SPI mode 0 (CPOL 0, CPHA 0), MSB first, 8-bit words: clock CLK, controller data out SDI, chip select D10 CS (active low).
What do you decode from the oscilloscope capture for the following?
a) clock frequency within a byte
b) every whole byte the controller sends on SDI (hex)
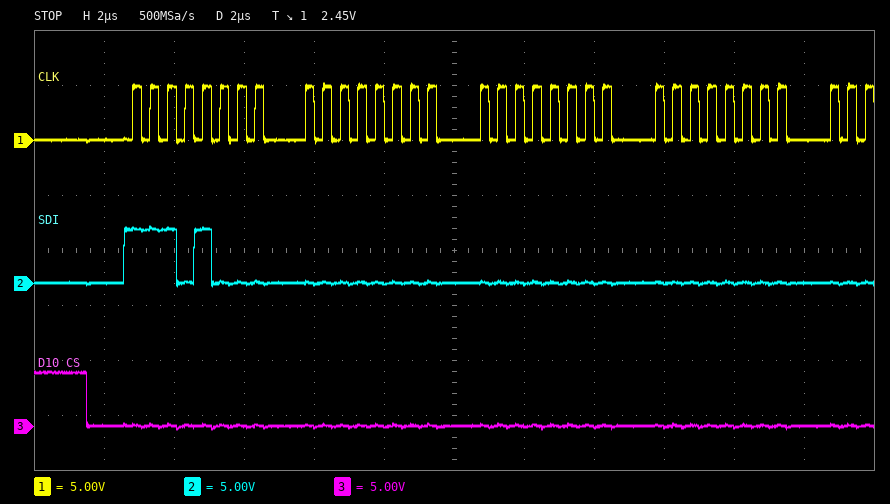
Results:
2 MHz
E8 00 00 00
